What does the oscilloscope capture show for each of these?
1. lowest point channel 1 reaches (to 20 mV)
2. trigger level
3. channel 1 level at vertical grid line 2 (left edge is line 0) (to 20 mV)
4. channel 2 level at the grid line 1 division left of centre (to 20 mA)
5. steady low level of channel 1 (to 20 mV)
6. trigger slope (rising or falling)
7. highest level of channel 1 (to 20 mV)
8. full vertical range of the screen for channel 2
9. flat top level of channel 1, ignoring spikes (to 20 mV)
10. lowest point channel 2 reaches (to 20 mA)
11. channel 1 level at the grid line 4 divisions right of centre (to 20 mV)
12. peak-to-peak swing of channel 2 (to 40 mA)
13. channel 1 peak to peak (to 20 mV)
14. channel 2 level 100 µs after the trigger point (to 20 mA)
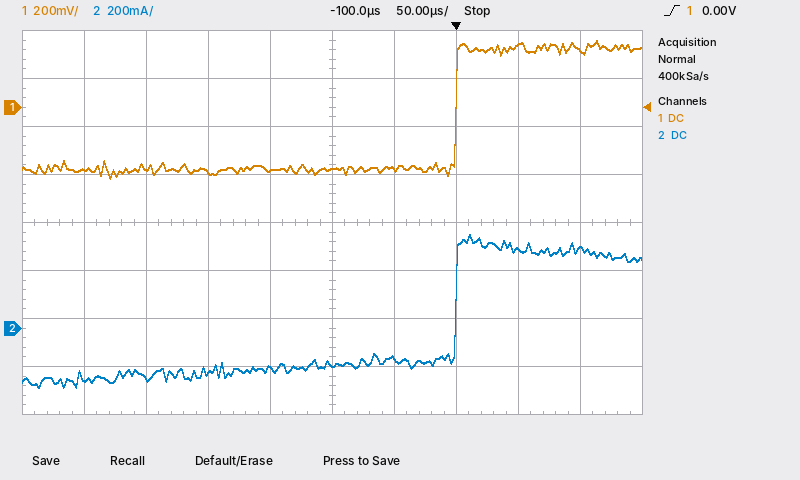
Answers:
-300 mV
0.00 V
-260 mV
-160 mA
-260 mV
rising
280 mV
1.6 A
240 mV
-240 mA
240 mV
640 mA
580 mV
340 mA
